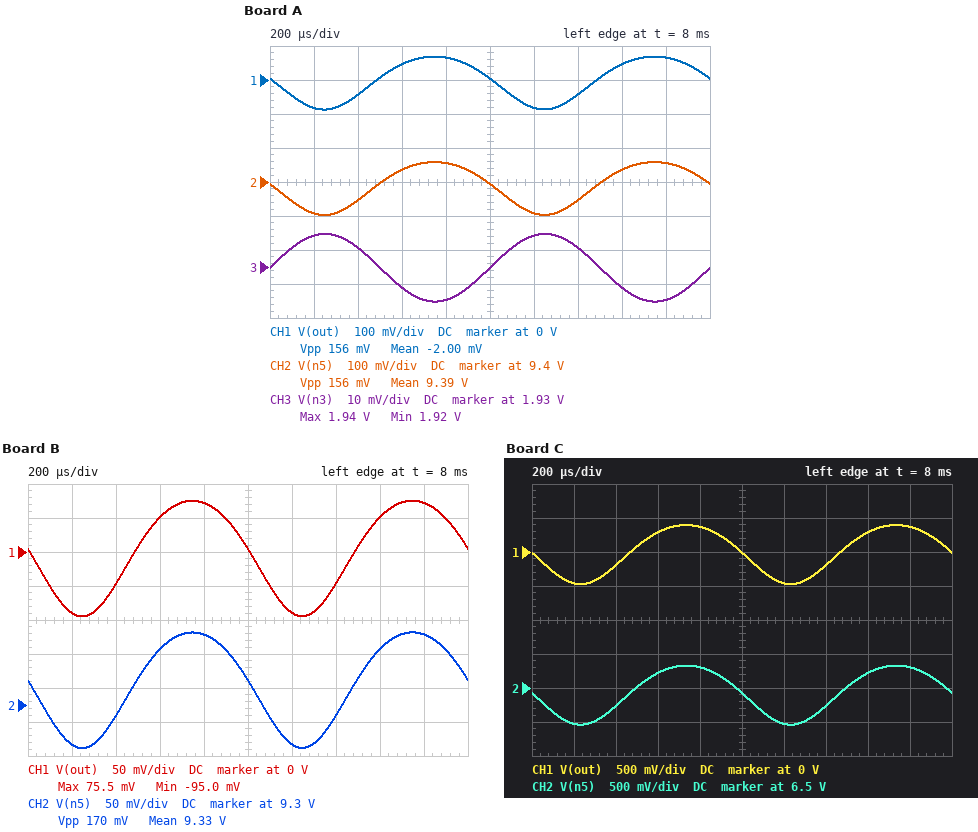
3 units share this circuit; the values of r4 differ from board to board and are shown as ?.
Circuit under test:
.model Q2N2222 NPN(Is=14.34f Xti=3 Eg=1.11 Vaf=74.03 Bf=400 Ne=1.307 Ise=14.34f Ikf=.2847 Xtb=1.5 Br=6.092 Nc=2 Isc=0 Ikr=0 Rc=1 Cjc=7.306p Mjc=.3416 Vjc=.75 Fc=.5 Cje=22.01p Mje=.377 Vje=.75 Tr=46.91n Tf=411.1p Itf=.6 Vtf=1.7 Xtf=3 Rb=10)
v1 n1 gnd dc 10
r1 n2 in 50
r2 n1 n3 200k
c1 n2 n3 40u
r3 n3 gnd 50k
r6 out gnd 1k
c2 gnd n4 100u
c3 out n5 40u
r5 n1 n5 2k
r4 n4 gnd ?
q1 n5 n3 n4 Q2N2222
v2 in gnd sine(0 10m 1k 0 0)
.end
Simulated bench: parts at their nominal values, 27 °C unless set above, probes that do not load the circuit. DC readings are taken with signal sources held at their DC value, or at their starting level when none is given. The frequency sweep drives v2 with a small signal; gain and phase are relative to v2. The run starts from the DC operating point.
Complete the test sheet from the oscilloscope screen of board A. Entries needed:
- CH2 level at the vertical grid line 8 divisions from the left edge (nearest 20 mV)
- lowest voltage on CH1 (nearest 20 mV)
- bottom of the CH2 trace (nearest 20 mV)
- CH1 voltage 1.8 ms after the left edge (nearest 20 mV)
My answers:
9.44 V
-80 mV
9.30 V
60 mV
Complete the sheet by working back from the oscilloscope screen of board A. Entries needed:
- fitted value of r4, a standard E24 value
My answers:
4.3 kΩ
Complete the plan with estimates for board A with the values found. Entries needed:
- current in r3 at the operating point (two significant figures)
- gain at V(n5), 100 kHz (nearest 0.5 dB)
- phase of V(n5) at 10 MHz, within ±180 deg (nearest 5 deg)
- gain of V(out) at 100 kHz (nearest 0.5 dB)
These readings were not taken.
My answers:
39 µA
18.0 dB
155 deg
18.0 dB
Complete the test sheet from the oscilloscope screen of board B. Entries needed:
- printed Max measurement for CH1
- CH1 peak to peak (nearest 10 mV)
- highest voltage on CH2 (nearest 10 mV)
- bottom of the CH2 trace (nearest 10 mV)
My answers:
75.5 mV
170 mV
9.41 V
9.24 V
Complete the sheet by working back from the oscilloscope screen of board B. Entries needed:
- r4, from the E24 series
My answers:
3.9 kΩ
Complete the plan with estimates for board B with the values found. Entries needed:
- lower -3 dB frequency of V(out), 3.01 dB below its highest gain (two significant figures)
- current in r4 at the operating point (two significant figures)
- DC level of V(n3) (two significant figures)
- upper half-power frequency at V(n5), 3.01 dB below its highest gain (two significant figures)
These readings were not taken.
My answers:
21 Hz
340 µA
1.9 V
28 MHz
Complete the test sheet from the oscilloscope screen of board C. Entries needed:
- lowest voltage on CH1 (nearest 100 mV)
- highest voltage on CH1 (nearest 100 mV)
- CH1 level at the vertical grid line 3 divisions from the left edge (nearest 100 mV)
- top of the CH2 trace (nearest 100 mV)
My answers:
-500 mV
400 mV
300 mV
6.8 V
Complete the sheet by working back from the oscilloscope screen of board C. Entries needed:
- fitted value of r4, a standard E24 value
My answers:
560 Ω
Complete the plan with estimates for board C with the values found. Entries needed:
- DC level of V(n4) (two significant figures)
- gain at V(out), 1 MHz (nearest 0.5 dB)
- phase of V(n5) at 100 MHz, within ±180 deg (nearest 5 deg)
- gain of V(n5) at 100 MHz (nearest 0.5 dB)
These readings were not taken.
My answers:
1.0 V
33.0 dB
75 deg
12.5 dB
